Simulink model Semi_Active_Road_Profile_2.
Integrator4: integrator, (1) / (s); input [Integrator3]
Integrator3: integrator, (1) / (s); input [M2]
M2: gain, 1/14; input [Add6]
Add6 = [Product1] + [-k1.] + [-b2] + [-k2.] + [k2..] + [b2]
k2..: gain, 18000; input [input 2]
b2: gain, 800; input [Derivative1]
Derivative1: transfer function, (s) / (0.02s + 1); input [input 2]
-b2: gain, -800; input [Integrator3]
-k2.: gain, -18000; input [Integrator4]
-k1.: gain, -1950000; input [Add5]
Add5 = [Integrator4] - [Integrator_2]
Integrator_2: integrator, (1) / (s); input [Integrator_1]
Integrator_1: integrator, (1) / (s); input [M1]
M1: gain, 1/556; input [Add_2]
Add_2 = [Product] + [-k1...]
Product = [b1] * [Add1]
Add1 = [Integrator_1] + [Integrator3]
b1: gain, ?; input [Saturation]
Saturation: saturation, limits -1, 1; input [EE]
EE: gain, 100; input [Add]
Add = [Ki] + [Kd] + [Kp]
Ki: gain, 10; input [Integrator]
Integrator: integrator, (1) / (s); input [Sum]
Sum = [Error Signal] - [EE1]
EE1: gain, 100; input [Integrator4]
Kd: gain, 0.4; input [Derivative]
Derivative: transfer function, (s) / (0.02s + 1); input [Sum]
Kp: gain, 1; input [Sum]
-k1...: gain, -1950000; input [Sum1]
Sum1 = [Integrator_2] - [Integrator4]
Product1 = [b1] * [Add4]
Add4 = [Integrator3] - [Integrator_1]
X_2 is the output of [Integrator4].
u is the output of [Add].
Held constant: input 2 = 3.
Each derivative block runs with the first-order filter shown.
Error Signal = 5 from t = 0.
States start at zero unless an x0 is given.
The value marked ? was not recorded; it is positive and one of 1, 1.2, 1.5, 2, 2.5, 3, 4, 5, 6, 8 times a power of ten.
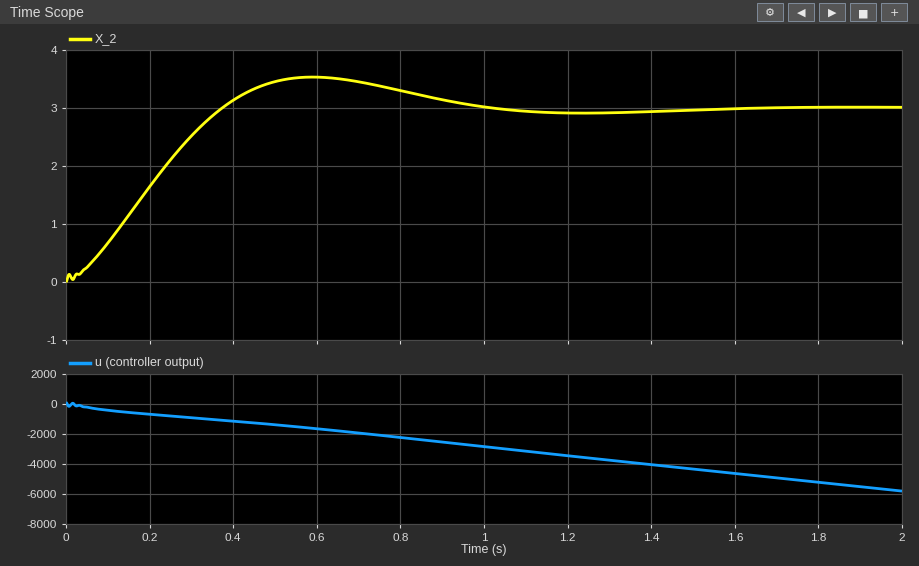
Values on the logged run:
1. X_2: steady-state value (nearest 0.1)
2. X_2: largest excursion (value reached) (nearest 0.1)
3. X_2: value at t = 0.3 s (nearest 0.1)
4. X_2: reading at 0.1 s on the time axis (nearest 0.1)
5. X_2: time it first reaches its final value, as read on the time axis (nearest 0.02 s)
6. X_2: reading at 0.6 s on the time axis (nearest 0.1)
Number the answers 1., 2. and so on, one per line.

1. 3.0
2. 3.5
3. 2.5
4. 0.7
5. 0.38 s
6. 3.5
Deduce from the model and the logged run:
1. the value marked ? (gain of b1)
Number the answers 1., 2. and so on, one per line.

1. 1200
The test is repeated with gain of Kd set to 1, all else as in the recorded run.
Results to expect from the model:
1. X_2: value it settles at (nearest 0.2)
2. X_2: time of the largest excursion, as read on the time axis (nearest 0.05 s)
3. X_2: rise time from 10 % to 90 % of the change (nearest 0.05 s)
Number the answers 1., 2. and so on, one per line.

1. 3.0
2. 0.60 s
3. 0.25 s
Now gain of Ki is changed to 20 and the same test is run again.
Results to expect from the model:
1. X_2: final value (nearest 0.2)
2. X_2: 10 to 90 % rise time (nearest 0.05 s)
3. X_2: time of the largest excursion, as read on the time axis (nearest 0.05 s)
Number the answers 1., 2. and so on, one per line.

1. 3.0
2. 0.25 s
3. 0.60 s
